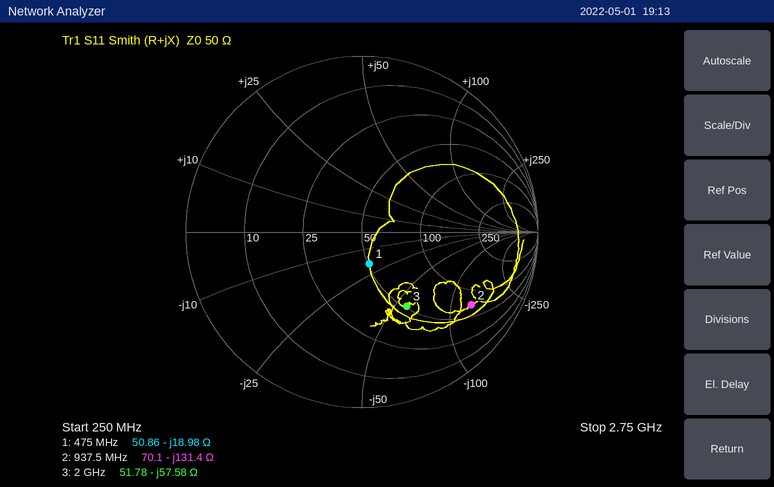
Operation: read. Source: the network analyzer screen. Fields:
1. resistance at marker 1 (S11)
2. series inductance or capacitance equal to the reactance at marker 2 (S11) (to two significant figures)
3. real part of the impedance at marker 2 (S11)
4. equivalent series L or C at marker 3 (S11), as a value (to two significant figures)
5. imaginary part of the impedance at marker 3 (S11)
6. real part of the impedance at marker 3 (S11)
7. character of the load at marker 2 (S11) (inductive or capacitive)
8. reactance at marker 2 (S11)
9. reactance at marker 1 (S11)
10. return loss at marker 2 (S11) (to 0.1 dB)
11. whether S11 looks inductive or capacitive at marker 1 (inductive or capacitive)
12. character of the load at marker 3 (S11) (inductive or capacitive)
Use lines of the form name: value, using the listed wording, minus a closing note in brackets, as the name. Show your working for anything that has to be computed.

resistance at marker 1: 50.86 Ω
series inductance or capacitance equal to the reactance at marker 2 (S11): C = 1/(2π × 937.5 MHz × 131.4 Ω) ≈ 1.3 pF
real part of the impedance at marker 2: 70.1 Ω
equivalent series L or C at marker 3 (S11), as a value: C = 1/(2π × 2 GHz × 57.58 Ω) ≈ 1.4 pF
imaginary part of the impedance at marker 3: -57.58 Ω
real part of the impedance at marker 3: 51.78 Ω
character of the load at marker 2 (S11): capacitive
reactance at marker 2: -131.4 Ω
reactance at marker 1: -18.98 Ω
return loss at marker 2 (S11): 2.5 dB
whether S11 looks inductive or capacitive at marker 1: capacitive
character of the load at marker 3 (S11): capacitive
